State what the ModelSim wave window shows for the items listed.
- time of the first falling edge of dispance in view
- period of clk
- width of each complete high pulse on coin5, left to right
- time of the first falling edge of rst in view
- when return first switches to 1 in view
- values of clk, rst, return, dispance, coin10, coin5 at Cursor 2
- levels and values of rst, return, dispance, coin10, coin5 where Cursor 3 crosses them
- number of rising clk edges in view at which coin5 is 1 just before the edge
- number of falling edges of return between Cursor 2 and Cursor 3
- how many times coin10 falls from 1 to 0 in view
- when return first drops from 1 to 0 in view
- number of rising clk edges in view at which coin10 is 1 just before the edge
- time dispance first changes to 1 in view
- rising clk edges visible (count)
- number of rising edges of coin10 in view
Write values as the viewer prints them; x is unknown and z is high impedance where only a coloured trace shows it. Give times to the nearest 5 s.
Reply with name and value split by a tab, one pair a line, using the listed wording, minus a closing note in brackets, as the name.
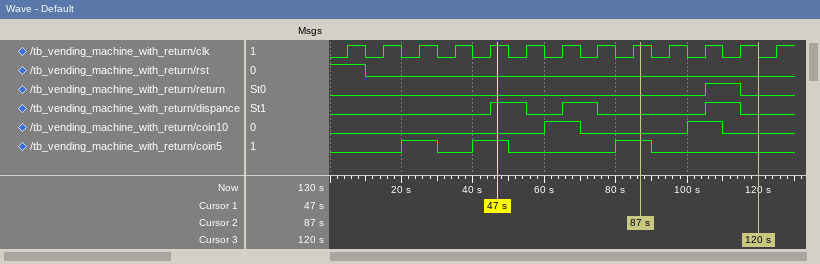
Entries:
time of the first falling edge of dispance in view	55 s
period of clk	10 s
width of each complete high pulse on coin5, left to right	10 s, 10 s, 10 s
time of the first falling edge of rst in view	10 s
when return first switches to 1 in view	105 s
values of clk, rst, return, dispance, coin10, coin5 at Cursor 2	clk=1, rst=0, return=0, dispance=0, coin10=0, coin5=1
levels and values of rst, return, dispance, coin10, coin5 where Cursor 3 crosses them	rst=0, return=0, dispance=0, coin10=0, coin5=0
number of rising clk edges in view at which coin5 is 1 just before the edge	3
number of falling edges of return between Cursor 2 and Cursor 3	1
how many times coin10 falls from 1 to 0 in view	2
when return first drops from 1 to 0 in view	115 s
number of rising clk edges in view at which coin10 is 1 just before the edge	2
time dispance first changes to 1 in view	45 s
rising clk edges visible	13
number of rising edges of coin10 in view	2
